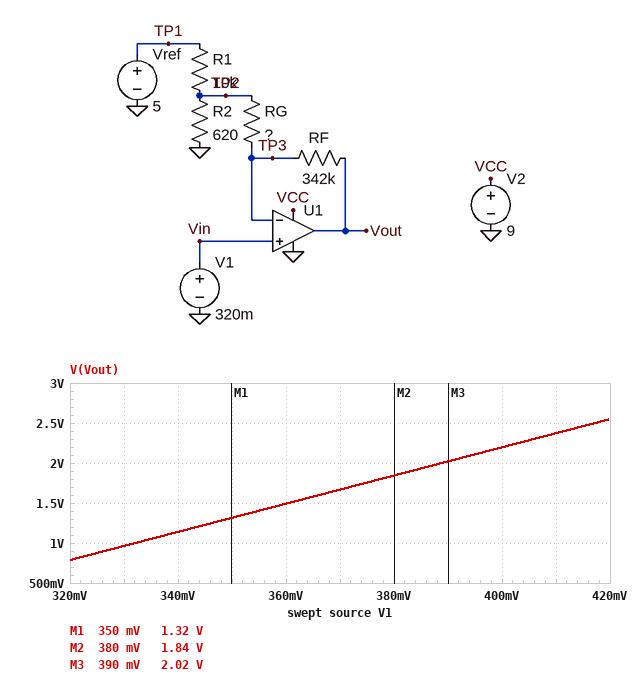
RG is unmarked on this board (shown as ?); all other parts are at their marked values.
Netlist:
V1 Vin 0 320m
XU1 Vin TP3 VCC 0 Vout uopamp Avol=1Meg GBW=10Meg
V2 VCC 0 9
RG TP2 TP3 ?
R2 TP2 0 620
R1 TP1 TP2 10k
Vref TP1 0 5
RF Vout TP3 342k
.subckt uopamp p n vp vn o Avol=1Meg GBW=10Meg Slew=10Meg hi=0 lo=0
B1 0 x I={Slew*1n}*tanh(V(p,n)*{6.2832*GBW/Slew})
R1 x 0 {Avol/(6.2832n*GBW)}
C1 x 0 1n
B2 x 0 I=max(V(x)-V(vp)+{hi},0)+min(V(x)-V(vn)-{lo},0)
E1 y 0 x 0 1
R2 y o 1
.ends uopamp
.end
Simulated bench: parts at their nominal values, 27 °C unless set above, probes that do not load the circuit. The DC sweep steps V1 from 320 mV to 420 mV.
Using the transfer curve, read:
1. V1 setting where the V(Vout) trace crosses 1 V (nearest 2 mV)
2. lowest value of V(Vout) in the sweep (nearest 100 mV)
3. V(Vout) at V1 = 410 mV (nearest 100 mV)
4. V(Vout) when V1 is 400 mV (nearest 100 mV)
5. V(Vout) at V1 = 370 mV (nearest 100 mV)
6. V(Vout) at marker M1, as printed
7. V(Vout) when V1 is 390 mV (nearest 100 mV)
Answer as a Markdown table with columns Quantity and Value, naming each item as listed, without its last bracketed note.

| Quantity | Value |
|---|---|
| V1 setting where the V(Vout) trace crosses 1 V | 332 mV |
| lowest value of V(Vout) in the sweep | 800 mV |
| V(Vout) at V1 = 410 mV | 2.4 V |
| V(Vout) when V1 is 400 mV | 2.2 V |
| V(Vout) at V1 = 370 mV | 1.7 V |
| V(Vout) at marker M1, as printed | 1.32 V |
| V(Vout) when V1 is 390 mV | 2.0 V |
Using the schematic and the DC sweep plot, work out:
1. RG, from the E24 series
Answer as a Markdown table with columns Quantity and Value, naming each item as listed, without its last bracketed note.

| Quantity | Value |
|---|---|
| RG, from the E24 series | 20 kΩ |
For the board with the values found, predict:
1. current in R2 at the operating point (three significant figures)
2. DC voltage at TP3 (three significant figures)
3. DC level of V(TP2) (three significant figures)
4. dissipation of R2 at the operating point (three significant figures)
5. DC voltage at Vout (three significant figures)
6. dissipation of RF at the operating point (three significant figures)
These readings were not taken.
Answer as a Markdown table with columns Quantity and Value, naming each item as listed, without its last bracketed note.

| Quantity | Value |
|---|---|
| current in R2 at the operating point | 472 µA |
| DC voltage at TP3 | 320 mV |
| DC level of V(TP2) | 293 mV |
| dissipation of R2 at the operating point | 138 µW |
| DC voltage at Vout | 787 mV |
| dissipation of RF at the operating point | 637 nW |
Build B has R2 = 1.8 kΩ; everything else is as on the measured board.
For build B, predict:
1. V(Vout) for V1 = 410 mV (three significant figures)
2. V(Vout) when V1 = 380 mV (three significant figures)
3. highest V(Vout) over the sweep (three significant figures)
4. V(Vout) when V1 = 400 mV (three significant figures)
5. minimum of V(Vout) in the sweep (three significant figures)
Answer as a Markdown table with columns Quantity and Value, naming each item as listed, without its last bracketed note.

| Quantity | Value |
|---|---|
| V(Vout) for V1 = 410 mV | -9.58 mV |
| V(Vout) when V1 = 380 mV | -9.71 mV |
| highest V(Vout) over the sweep | -9.53 mV |
| V(Vout) when V1 = 400 mV | -9.63 mV |
| minimum of V(Vout) in the sweep | -9.86 mV |
